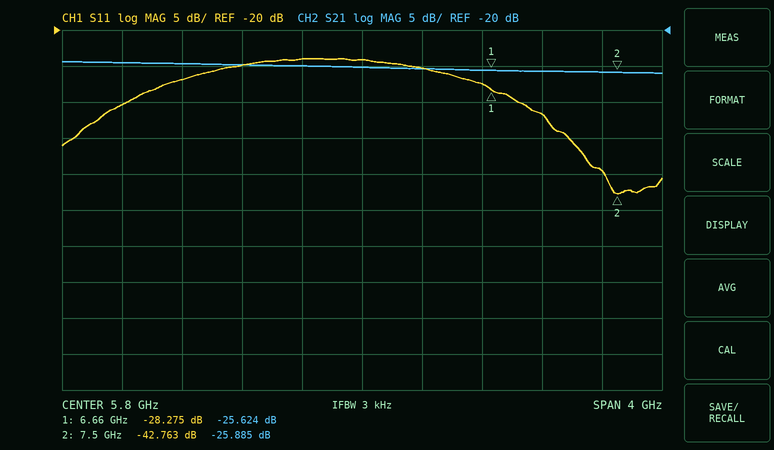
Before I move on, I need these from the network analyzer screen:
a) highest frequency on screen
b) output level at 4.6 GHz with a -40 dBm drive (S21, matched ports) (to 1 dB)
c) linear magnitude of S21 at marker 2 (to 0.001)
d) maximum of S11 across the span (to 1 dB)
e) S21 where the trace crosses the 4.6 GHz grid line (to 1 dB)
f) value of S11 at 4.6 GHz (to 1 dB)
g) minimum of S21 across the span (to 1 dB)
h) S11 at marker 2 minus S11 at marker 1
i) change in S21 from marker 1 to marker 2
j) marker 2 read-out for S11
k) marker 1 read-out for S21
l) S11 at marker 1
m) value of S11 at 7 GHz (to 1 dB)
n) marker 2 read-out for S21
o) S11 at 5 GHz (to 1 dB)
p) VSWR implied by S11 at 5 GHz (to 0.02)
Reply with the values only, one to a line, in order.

7.8 GHz
-65 dBm
0.051
-24 dB
-25 dB
-27 dB
-26 dB
-14.488 dB
-0.261 dB
-42.763 dB
-25.624 dB
-28.275 dB
-32 dB
-25.885 dB
-25 dB
1.12
